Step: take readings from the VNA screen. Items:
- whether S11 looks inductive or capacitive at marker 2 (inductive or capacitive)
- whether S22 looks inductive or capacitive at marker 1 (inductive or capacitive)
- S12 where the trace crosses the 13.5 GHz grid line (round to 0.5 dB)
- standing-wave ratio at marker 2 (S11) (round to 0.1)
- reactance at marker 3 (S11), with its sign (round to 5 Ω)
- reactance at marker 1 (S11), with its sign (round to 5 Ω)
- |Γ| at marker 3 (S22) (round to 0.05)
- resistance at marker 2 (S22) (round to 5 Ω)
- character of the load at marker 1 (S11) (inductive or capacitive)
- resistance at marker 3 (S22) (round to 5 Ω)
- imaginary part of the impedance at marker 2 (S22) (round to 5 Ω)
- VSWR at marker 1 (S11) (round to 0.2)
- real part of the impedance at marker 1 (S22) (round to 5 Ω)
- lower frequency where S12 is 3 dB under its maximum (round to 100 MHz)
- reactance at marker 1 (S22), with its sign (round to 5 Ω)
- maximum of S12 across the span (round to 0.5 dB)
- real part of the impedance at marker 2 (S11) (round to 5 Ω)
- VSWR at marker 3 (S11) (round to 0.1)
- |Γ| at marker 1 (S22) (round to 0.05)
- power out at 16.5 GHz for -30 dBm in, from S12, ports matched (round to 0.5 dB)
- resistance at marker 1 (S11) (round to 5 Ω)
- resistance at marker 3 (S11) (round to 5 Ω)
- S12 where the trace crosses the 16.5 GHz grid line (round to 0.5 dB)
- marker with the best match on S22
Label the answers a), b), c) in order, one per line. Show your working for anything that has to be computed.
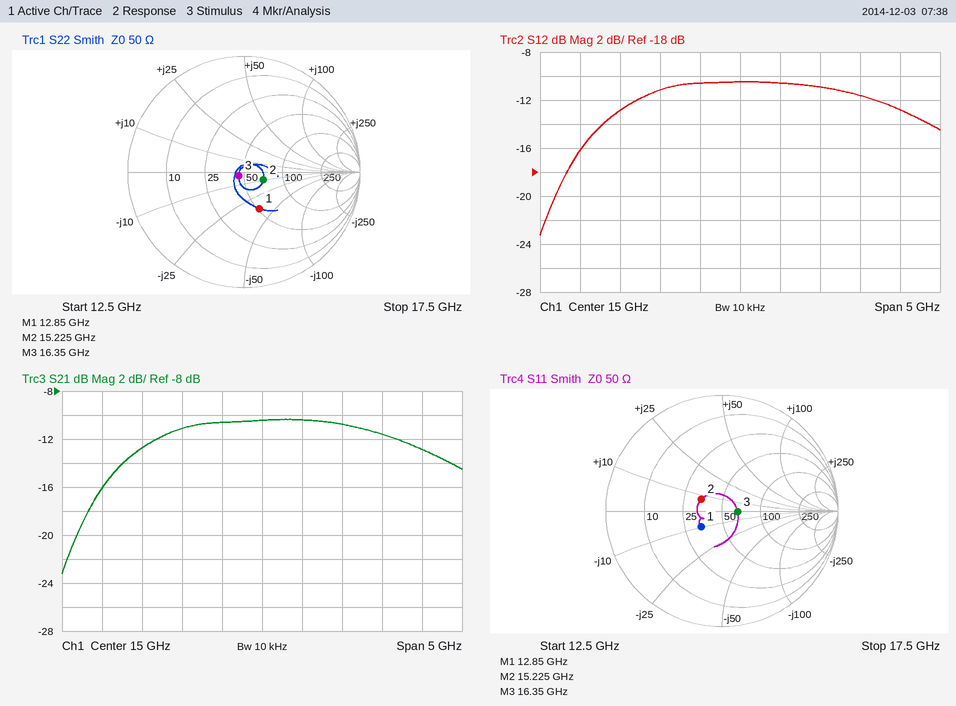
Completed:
a) inductive
b) capacitive
c) -13.0 dB
d) 1.5
e) 0 Ω
f) -10 Ω
g) 0.05
h) 70 Ω
i) capacitive
j) 45 Ω
k) -10 Ω
l) 1.6
m) 50 Ω
n) 13.4 GHz
o) -35 Ω
p) -10.5 dB
q) 35 Ω
r) 1.3
s) 0.35
t) -30 dBm + (-11.5 dB) = -41.5 dBm
u) 35 Ω
v) 65 Ω
w) -11.5 dB
x) marker 3
